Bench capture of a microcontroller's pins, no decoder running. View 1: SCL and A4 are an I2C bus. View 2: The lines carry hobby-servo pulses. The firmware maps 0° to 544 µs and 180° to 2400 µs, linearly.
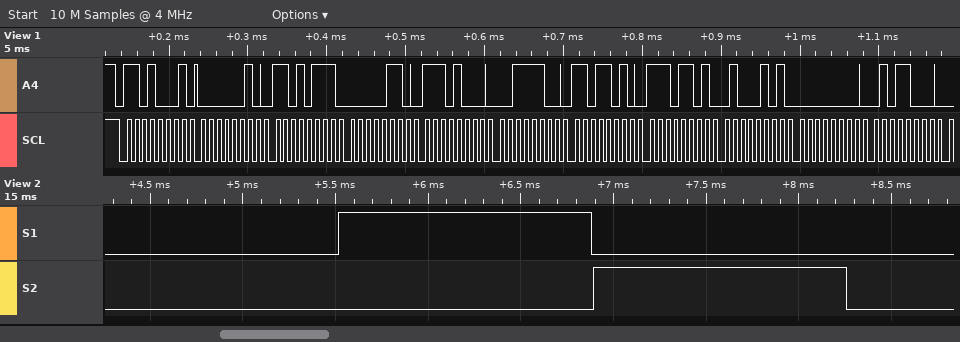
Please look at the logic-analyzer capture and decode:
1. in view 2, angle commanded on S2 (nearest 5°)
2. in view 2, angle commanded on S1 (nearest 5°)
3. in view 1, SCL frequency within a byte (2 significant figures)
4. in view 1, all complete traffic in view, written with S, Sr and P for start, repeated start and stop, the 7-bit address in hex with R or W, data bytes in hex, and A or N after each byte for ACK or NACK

80°
80°
100 kHz
S 68R A 02 A D7 A 06 A E8 A 3C A DA A ED A 45 A 00 A 58 A
